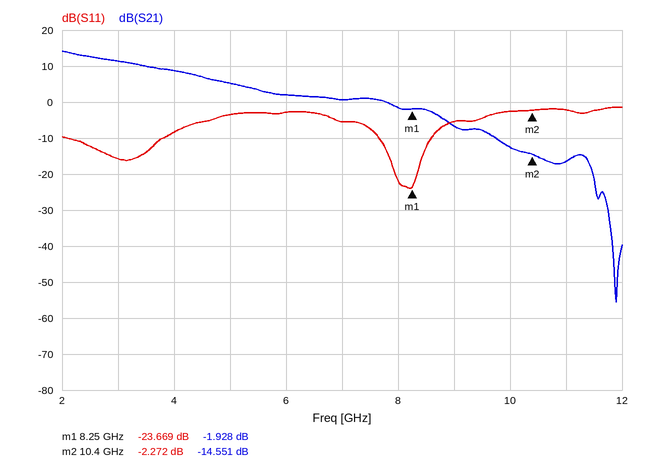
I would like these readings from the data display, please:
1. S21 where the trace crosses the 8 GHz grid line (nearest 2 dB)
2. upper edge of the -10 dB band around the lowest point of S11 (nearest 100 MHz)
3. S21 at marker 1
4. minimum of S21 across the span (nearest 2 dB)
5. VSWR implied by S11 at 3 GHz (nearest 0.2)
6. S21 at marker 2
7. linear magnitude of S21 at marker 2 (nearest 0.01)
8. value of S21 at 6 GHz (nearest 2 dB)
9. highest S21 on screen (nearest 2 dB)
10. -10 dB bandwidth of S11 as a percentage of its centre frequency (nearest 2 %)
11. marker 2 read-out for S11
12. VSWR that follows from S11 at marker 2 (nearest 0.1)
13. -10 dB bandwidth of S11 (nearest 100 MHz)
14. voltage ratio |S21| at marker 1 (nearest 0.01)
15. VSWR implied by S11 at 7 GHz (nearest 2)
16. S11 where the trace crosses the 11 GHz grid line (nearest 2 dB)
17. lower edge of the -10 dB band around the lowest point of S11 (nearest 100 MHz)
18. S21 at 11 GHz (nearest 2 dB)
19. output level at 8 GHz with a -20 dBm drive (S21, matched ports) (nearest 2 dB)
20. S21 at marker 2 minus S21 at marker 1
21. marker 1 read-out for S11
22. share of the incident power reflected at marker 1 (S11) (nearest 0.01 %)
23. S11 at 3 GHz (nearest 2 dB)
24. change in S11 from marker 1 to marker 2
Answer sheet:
-2 dB
8.6 GHz
-1.928 dB
-56 dB
1.4
-14.551 dB
0.19
2 dB
14 dB
12 %
-2.272 dB
7.7
900 MHz
0.80
4
-2 dB
7.7 GHz
-16 dB
-22 dBm
-12.623 dB
-23.669 dB
0.43 %
-16 dB
21.397 dB
